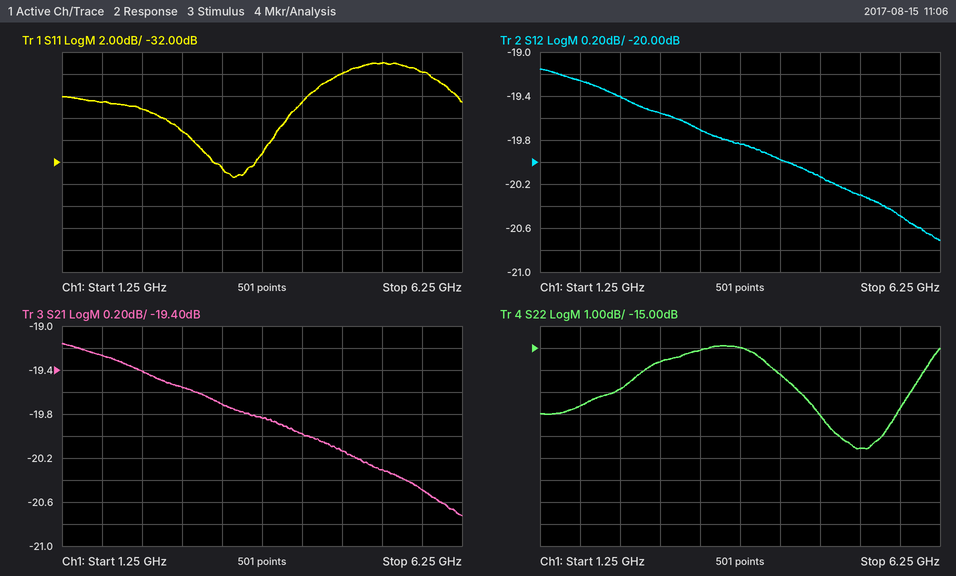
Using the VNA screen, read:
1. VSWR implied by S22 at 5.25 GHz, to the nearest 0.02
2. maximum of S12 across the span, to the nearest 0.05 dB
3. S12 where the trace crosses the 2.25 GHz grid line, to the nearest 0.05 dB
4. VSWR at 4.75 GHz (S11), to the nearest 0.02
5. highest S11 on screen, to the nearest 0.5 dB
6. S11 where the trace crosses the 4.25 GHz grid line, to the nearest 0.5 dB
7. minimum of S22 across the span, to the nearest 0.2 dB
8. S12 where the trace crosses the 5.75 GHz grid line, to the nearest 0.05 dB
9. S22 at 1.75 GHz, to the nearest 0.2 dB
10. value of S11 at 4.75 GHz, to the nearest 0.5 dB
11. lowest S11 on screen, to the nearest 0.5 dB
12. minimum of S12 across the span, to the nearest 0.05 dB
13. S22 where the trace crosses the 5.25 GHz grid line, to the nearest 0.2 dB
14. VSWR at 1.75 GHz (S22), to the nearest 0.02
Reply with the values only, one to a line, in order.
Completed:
1.24
-19.15 dB
-19.40 dB
1.14
-23.0 dB
-26.5 dB
-19.6 dB
-20.50 dB
-17.6 dB
-24.0 dB
-33.5 dB
-20.70 dB
-19.6 dB
1.30
